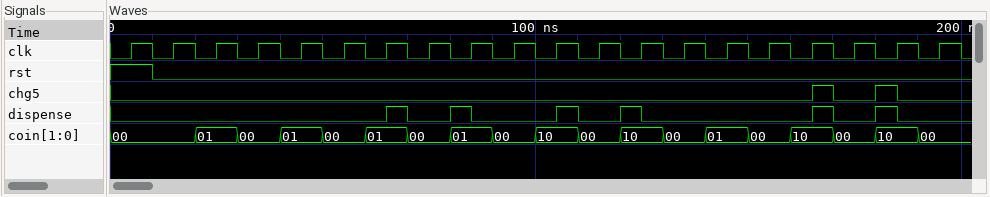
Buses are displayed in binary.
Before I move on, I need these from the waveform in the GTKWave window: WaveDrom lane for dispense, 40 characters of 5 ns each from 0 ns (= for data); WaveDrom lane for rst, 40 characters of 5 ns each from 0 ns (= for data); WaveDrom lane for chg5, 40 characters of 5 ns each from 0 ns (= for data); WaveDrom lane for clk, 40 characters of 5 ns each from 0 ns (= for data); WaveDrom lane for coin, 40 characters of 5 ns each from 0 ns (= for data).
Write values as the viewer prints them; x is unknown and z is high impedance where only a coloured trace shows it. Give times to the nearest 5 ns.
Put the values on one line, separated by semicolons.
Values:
{name: 'dispense', wave: '0............10.10...10.10.......10.10..'}; {name: 'rst', wave: '1.0.....................................'}; {name: 'chg5', wave: '0................................10.10..'}; {name: 'clk', wave: '0101010101010101010101010101010101010101'}; {name: 'coin', wave: '=...=.=.=.=.=.=.=.=.=.=.=.=.=.=.=.=.=.=.', data: '00 01 00 01 00 01 00 01 00 10 00 10 00 01 00 10 00 10 00'}
